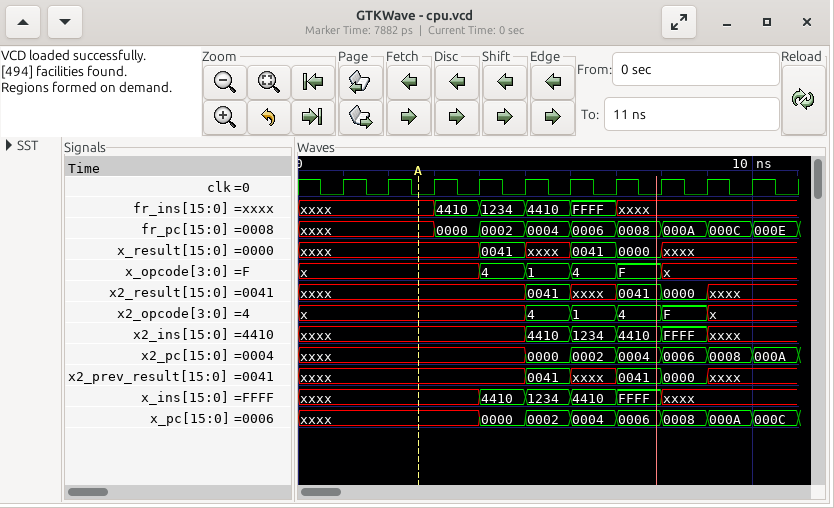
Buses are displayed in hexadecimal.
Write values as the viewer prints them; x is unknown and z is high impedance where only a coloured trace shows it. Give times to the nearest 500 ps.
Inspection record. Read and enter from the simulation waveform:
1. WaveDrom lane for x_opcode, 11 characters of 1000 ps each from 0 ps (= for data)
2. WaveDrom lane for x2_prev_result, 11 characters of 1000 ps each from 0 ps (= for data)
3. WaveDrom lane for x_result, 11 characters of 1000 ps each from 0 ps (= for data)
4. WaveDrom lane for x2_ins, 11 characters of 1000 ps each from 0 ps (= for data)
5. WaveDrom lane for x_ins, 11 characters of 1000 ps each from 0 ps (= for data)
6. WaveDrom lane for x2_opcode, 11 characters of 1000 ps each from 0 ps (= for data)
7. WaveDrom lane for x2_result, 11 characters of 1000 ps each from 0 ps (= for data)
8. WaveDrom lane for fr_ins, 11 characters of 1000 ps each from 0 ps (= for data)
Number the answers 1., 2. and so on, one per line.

1. {name: 'x_opcode', wave: 'x...====x..', data: '4 1 4 F'}
2. {name: 'x2_prev_result', wave: 'x....=x==x.', data: '0041 0041 0000'}
3. {name: 'x_result', wave: 'x...=x==x..', data: '0041 0041 0000'}
4. {name: 'x2_ins', wave: 'x....====x.', data: '4410 1234 4410 FFFF'}
5. {name: 'x_ins', wave: 'x...====x..', data: '4410 1234 4410 FFFF'}
6. {name: 'x2_opcode', wave: 'x....====x.', data: '4 1 4 F'}
7. {name: 'x2_result', wave: 'x....=x==x.', data: '0041 0041 0000'}
8. {name: 'fr_ins', wave: 'x..====x...', data: '4410 1234 4410 FFFF'}
